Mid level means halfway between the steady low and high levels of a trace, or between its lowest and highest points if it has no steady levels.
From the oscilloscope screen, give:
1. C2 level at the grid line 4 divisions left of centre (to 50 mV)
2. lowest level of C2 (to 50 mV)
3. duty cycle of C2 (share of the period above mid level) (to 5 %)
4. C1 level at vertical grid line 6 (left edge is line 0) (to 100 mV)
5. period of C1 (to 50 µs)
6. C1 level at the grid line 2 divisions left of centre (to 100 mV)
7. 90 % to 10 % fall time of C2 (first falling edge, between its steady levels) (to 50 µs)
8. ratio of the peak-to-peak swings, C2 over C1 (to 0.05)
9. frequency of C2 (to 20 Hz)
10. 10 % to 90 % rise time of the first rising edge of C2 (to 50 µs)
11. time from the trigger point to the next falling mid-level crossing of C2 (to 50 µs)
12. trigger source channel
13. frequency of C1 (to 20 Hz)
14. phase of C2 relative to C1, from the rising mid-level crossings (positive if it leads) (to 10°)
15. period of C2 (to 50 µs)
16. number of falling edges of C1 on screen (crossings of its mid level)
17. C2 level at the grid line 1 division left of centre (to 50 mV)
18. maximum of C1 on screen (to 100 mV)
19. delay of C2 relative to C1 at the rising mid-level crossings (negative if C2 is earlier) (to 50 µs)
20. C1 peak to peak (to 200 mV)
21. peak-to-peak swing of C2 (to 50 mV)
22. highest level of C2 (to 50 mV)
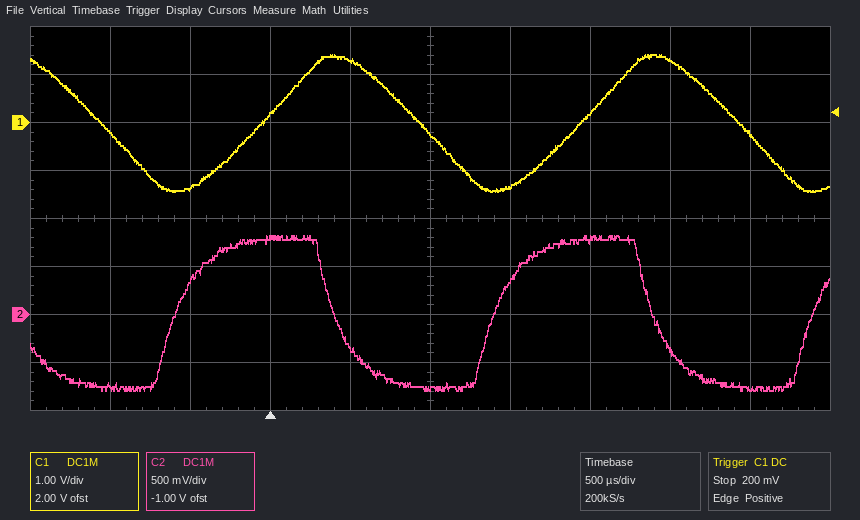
-750 mV
-800 mV
50 %
-1.3 V
2.00 ms
200 mV
350 µs
0.55
500 Hz
350 µs
400 µs
C1
500 Hz
+100°
2.00 ms
3
-350 mV
1.4 V
-550 µs
2.8 V
1.60 V
800 mV
